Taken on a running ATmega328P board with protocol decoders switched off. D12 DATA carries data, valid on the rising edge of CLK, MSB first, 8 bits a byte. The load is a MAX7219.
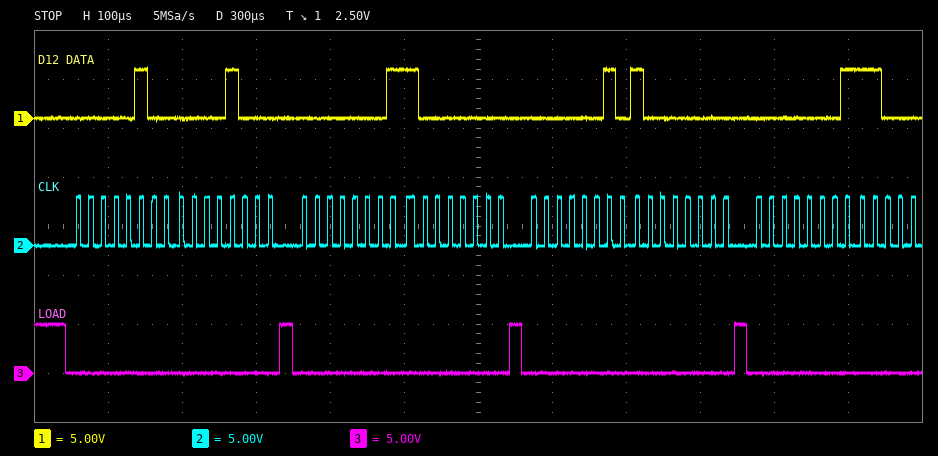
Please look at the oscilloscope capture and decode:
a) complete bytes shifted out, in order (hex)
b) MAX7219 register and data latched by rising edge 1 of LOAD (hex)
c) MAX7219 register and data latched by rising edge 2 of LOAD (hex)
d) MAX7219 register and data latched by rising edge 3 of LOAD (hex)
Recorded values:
04 08 01 80 02 80 01
register 0x4, data 0x08
register 0x1, data 0x80
register 0x2, data 0x80
